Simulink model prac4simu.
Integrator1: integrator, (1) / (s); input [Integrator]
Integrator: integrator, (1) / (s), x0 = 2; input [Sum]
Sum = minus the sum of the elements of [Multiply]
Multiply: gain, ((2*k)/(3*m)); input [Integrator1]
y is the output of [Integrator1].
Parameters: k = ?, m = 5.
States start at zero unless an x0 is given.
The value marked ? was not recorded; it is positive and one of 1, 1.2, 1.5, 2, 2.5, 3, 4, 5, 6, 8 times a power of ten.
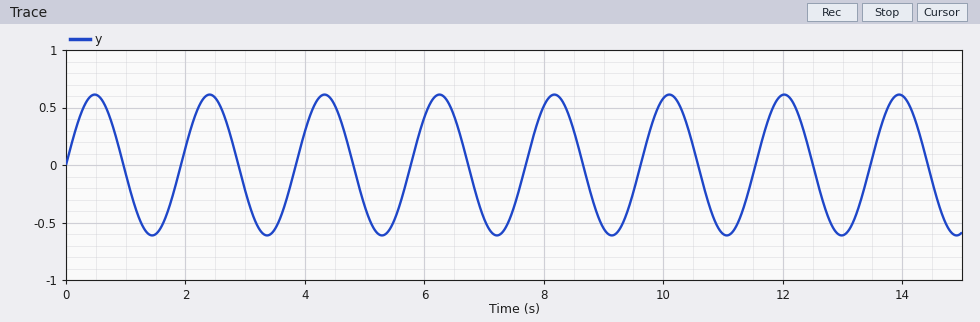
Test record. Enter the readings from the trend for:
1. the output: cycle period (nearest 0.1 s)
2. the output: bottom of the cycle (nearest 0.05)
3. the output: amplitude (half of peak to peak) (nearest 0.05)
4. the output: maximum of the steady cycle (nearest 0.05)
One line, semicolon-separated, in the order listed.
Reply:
1.9 s; -0.60; 0.60; 0.60
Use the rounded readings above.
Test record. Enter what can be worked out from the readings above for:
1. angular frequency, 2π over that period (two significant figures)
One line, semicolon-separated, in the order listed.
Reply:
3.3 rad/s
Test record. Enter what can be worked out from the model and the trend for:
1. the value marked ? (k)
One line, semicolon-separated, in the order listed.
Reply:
80
